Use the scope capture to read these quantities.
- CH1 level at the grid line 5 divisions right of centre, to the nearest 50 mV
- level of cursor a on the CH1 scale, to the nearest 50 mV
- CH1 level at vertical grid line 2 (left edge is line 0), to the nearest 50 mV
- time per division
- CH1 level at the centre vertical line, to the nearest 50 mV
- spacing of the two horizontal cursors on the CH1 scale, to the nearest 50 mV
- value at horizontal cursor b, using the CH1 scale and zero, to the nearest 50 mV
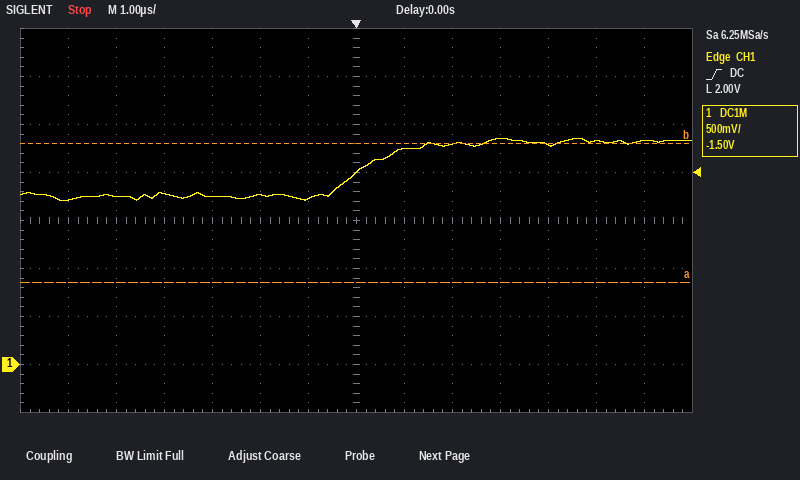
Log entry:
2.35 V
850 mV
1.75 V
1 µs
2.00 V
1.45 V
2.30 V
